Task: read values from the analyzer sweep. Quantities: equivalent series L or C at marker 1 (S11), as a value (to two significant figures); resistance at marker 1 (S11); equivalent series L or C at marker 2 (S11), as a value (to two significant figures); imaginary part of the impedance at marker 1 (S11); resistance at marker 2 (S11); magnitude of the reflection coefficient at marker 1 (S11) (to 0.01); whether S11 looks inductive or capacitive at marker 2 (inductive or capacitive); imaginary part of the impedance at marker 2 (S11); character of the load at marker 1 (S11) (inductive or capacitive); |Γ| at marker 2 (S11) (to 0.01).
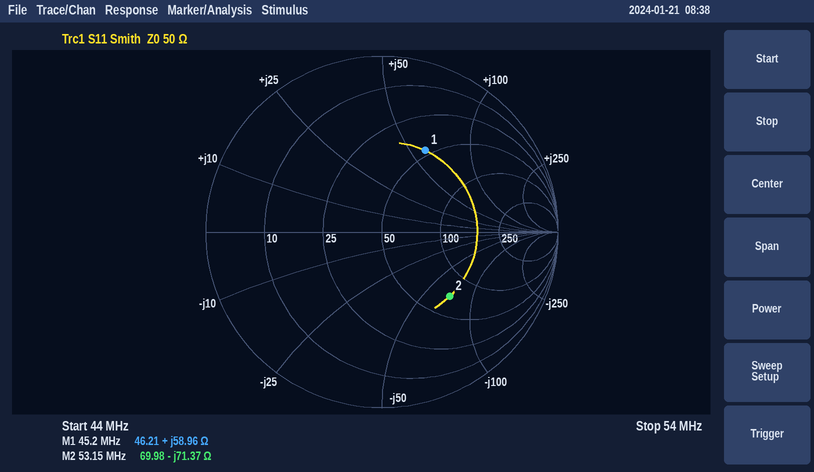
210 nH
46.21 Ω
42 pF
+58.96 Ω
69.98 Ω
0.52
capacitive
-71.37 Ω
inductive
0.53
